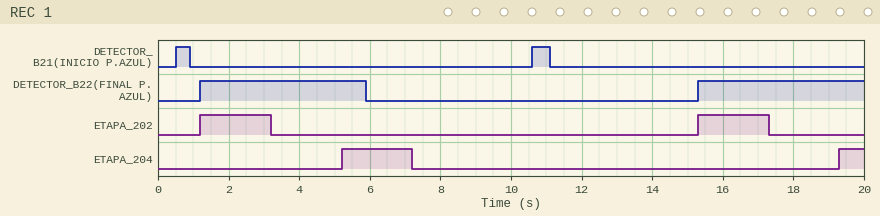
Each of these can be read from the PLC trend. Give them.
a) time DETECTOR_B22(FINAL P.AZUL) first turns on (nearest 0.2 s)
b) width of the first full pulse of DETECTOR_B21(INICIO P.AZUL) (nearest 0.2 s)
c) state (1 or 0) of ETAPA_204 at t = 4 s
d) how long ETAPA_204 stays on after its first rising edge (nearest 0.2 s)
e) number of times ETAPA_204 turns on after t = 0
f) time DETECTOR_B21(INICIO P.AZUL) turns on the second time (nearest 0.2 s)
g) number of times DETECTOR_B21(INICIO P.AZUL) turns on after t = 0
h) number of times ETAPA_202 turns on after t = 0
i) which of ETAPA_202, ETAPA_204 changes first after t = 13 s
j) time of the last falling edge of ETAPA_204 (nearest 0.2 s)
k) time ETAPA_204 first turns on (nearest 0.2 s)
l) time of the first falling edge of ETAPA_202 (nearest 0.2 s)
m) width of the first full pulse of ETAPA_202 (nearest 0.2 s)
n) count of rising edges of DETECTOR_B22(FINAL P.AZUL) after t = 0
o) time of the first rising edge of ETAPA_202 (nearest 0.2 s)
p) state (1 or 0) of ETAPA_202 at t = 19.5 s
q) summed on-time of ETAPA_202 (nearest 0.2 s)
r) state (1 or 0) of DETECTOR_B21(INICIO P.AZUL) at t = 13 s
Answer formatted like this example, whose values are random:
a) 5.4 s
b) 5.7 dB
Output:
a) 1.2 s
b) 0.4 s
c) 0
d) 2.0 s
e) 2
f) 10.6 s
g) 2
h) 2
i) ETAPA_202
j) 7.2 s
k) 5.2 s
l) 3.2 s
m) 2.0 s
n) 2
o) 1.2 s
p) 0
q) 4.0 s
r) 0
